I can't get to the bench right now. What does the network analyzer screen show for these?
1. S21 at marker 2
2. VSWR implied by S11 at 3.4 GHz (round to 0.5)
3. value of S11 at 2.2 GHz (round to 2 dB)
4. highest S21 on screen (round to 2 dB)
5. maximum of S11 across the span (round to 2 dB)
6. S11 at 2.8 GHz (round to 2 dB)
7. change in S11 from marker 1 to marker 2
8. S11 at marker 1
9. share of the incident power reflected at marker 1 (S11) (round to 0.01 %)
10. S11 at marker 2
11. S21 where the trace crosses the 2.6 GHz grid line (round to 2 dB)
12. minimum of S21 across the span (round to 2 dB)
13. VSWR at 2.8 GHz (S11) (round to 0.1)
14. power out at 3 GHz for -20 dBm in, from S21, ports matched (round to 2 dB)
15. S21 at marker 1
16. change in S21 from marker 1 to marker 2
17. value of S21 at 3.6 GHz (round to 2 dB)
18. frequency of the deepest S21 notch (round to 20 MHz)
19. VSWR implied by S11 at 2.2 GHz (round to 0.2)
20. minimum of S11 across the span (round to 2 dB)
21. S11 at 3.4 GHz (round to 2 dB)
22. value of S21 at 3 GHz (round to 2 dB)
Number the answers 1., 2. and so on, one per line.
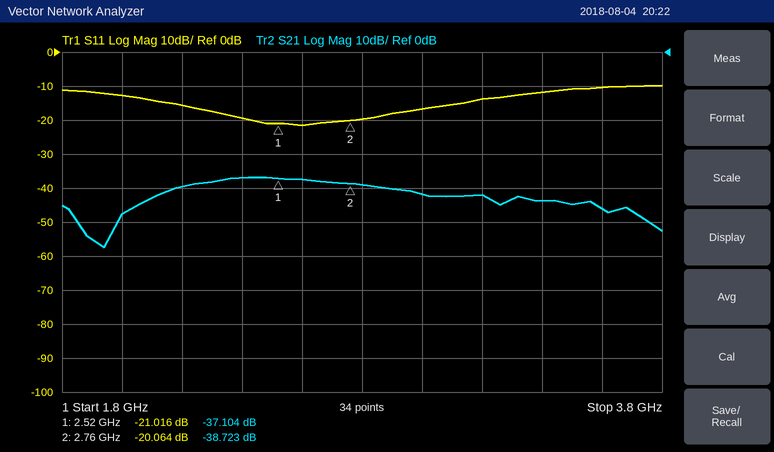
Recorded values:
1. -38.723 dB
2. 1.5
3. -16 dB
4. -36 dB
5. -10 dB
6. -20 dB
7. 0.952 dB
8. -21.016 dB
9. 0.79 %
10. -20.064 dB
11. -38 dB
12. -58 dB
13. 1.2
14. -62 dBm
15. -37.104 dB
16. -1.619 dB
17. -46 dB
18. 1.94 GHz
19. 1.4
20. -22 dB
21. -12 dB
22. -42 dB
